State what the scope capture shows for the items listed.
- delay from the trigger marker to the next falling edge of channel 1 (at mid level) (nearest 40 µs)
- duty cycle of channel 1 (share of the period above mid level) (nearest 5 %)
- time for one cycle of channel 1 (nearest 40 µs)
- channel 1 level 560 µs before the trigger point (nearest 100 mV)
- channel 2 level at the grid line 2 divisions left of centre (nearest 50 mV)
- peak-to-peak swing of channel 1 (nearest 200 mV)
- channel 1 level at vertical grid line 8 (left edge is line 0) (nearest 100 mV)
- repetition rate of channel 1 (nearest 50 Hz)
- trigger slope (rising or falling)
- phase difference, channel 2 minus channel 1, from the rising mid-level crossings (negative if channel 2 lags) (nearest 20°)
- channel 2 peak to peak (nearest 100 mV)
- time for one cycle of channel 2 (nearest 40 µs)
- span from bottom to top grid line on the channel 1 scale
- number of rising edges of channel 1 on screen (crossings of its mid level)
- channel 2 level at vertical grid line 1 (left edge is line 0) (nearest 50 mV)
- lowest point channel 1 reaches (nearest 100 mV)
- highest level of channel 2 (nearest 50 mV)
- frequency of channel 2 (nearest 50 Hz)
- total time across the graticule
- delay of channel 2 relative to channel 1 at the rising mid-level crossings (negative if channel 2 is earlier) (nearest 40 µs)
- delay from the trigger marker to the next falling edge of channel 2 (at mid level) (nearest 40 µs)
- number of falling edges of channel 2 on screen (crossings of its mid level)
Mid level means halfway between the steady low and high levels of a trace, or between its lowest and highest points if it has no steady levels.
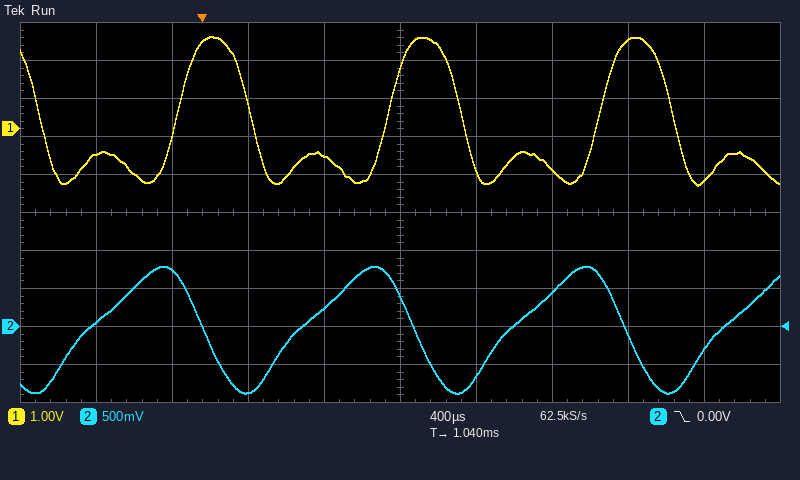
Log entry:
240 µs
35 %
1.12 ms
-700 mV
-850 mV
4.0 V
2.3 V
900 Hz
falling
+160°
1.70 V
1.12 ms
10 V
3
50 mV
-1.5 V
800 mV
900 Hz
4 ms
-480 µs
1.12 ms
3
